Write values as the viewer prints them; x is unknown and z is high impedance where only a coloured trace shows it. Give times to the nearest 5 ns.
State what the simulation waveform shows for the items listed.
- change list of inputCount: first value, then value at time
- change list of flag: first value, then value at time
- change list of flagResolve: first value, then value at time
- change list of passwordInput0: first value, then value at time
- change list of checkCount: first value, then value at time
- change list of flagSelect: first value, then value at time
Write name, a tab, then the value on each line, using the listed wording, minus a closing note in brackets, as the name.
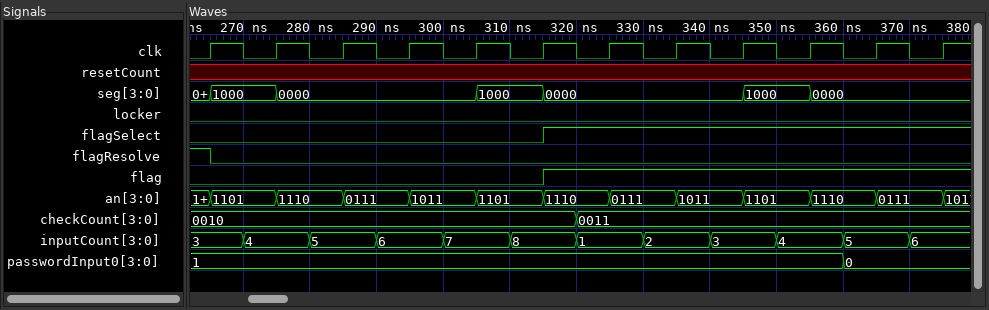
change list of inputCount: first value, then value at time	3, 4 at 270 ns, 5 at 280 ns, 6 at 290 ns, 7 at 300 ns, 8 at 310 ns, 1 at 320 ns, 2 at 330 ns, 3 at 340 ns, 4 at 350 ns, 5 at 360 ns, 6 at 370 ns
change list of flag: first value, then value at time	0, 1 at 315 ns
change list of flagResolve: first value, then value at time	1, 0 at 265 ns
change list of passwordInput0: first value, then value at time	1, 0 at 360 ns
change list of checkCount: first value, then value at time	0010, 0011 at 320 ns
change list of flagSelect: first value, then value at time	0, 1 at 315 ns
